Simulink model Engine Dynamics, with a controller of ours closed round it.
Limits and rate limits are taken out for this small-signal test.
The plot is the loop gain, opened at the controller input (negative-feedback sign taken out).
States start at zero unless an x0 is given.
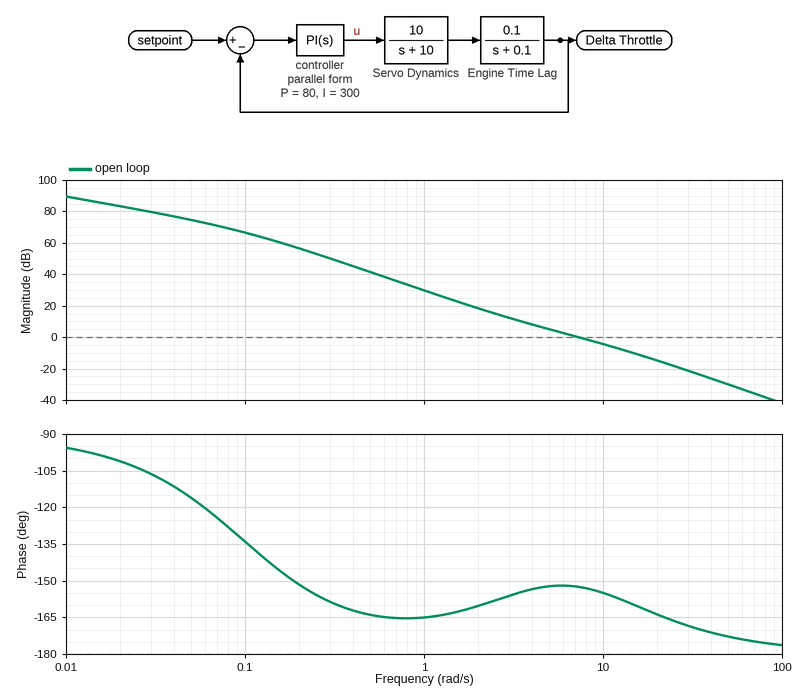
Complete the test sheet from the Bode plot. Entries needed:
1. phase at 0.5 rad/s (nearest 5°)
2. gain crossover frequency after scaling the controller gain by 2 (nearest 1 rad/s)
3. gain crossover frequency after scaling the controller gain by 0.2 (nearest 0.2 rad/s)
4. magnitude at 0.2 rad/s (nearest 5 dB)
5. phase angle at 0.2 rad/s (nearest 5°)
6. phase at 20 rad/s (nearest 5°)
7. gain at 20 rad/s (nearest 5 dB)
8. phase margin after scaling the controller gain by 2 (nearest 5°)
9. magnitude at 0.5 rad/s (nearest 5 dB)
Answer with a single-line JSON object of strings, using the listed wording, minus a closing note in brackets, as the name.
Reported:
{"phase at 0.5 rad/s": "-165°", "gain crossover frequency after scaling the controller gain by 2": "11 rad/s", "gain crossover frequency after scaling the controller gain by 0.2": "2.6 rad/s", "magnitude at 0.2 rad/s": "55 dB", "phase angle at 0.2 rad/s": "-150°", "phase at 20 rad/s": "-165°", "gain at 20 rad/s": "-15 dB", "phase margin after scaling the controller gain by 2": "25°", "magnitude at 0.5 rad/s": "40 dB"}
